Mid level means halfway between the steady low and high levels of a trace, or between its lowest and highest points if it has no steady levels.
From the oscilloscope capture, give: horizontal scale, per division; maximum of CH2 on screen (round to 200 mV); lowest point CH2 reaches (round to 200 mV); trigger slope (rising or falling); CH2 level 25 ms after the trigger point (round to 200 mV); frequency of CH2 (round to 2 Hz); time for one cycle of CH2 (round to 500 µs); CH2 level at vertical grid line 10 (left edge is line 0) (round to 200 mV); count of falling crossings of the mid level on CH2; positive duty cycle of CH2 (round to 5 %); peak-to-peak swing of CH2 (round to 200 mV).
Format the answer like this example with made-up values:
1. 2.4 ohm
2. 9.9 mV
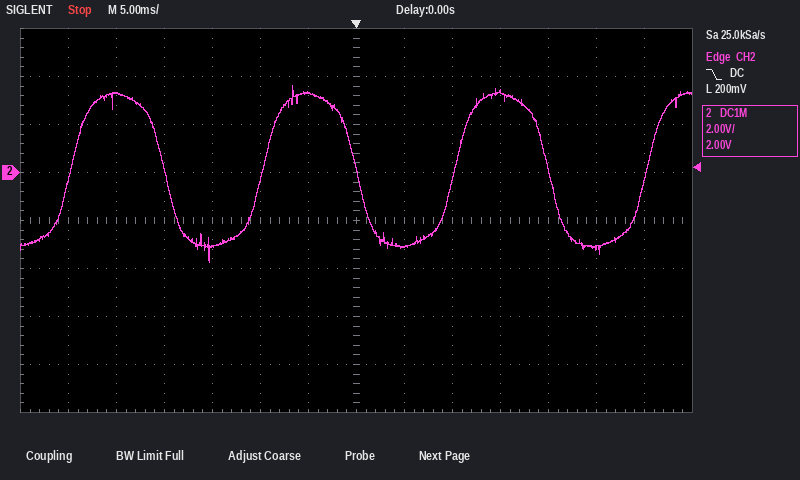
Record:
1. 5 ms
2. 3.6 V
3. -3.8 V
4. falling
5. -3.2 V
6. 50 Hz
7. 20.0 ms
8. 3.4 V
9. 3
10. 50 %
11. 7.4 V
